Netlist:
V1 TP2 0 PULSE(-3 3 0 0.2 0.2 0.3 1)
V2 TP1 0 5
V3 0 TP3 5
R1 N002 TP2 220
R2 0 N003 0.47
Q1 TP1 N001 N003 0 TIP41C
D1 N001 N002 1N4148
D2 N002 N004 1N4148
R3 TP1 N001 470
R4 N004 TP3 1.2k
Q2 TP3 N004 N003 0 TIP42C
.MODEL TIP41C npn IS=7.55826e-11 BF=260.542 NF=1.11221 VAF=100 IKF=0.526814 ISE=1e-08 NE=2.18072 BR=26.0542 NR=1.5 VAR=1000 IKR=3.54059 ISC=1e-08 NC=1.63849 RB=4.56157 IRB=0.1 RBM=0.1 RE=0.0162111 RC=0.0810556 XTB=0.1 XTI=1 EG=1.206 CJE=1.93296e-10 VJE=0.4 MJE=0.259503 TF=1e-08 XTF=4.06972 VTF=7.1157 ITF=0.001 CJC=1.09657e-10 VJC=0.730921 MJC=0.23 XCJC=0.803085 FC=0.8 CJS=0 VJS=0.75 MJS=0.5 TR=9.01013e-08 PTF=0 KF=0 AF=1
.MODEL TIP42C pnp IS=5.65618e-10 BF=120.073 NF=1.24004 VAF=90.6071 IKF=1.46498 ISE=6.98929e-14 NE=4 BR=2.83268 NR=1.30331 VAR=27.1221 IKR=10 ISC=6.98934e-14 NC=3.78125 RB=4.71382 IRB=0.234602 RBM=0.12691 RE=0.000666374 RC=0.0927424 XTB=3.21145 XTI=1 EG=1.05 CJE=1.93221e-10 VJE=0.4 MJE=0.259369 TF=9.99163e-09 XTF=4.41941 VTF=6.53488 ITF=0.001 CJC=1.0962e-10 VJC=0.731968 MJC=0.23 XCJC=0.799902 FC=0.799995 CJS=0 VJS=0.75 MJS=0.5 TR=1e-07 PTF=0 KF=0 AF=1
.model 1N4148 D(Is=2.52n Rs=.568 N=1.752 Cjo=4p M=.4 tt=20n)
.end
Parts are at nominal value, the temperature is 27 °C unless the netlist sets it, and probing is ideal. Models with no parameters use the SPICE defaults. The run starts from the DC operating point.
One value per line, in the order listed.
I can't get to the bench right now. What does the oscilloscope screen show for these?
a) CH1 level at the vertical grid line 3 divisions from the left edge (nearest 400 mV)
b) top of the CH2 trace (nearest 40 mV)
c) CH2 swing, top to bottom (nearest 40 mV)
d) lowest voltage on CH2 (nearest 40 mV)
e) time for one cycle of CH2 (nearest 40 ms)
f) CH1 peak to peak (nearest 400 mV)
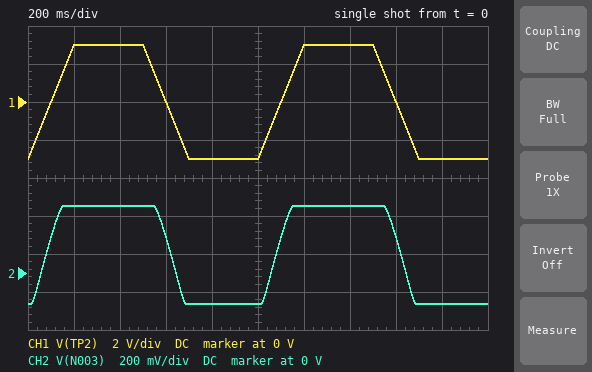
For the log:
0 V
360 mV
520 mV
-160 mV
1.00 s
6.0 V
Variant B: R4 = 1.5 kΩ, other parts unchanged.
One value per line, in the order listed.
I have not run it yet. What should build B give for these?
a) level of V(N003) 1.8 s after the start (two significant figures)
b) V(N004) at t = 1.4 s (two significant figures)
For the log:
-140 mV
1.4 V
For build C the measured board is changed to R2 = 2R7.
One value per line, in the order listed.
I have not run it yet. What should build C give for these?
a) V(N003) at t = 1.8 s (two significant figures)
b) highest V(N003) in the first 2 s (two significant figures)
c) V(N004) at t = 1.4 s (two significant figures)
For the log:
-660 mV
1.5 V
1.2 V
